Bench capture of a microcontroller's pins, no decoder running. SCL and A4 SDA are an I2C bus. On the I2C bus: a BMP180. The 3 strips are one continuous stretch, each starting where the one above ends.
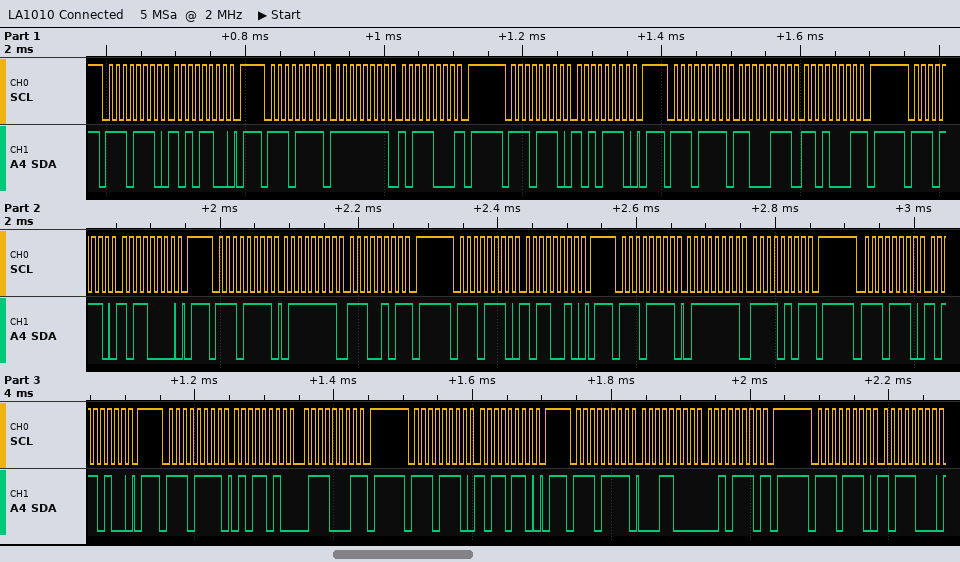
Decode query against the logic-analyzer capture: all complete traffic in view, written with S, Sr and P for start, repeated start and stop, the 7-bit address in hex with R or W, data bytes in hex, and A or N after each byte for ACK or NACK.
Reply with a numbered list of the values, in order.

1. S 77W A AC A P S 77R A FF A B8 N P S 77W A AE A P S 77R A C7 A D1 N P S 77W A B0 A P S 77R A 7F A E5 N P S 77W A B2 A P S 77R A 7F A F5 N P S 77W A B4 A P S 77R A 5A A 71 N P S 77W A B6 A P S 77R A 18 A 2E N P S 77W A B8 A
